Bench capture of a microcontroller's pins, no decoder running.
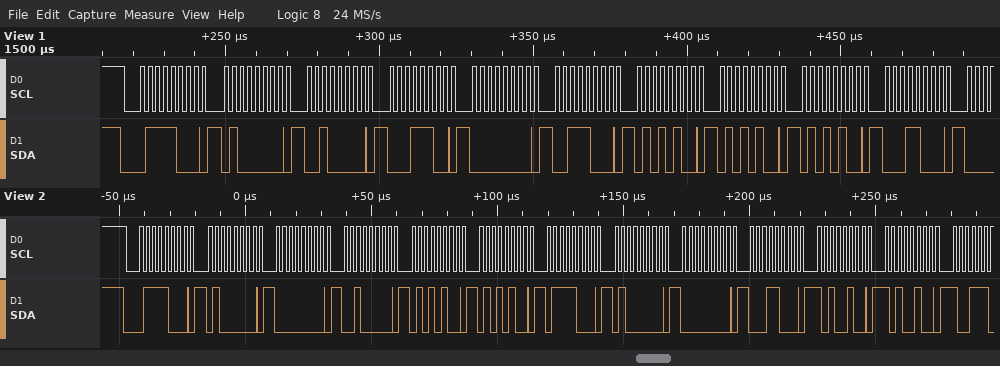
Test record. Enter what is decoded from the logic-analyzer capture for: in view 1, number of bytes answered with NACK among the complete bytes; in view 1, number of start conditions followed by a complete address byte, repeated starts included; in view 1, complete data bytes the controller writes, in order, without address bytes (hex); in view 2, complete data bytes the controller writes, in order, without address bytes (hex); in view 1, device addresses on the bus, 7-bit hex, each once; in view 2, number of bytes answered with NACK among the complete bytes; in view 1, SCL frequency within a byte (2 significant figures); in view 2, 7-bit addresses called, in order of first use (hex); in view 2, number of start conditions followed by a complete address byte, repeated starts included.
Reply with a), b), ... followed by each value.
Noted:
a) 0
b) 1
c) 40 20 1C 00 38 54 54 54 18
d) 40 00 20 54 54 78 40 00 18 A4 A4
e) 0x3C
f) 0
g) 400 kHz
h) 0x3C
i) 1
